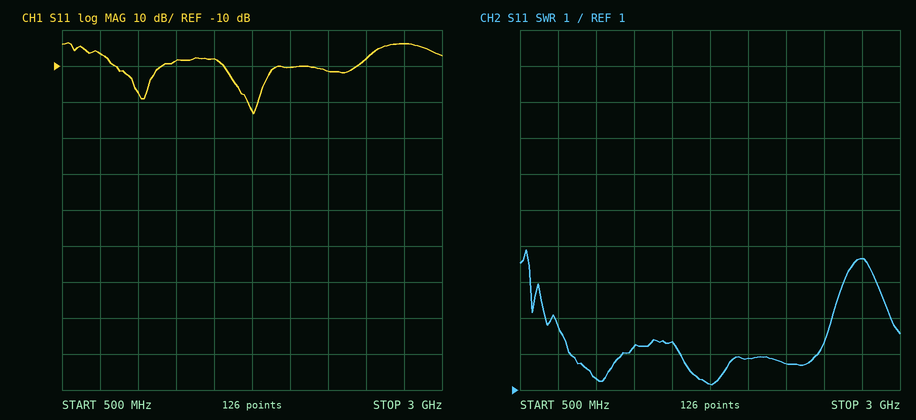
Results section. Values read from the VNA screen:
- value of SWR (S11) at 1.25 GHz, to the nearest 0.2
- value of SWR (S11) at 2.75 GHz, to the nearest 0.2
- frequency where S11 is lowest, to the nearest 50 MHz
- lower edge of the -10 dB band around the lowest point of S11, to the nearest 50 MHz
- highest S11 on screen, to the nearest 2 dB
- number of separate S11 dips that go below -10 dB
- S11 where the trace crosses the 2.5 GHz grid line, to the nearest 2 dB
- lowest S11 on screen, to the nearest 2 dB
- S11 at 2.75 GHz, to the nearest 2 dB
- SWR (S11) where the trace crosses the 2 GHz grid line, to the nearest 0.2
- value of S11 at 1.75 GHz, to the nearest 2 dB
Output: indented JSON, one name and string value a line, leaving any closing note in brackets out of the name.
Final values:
{
  "value of SWR (S11) at 1.25 GHz, to the nearest 0.2": "2.2",
  "value of SWR (S11) at 2.75 GHz, to the nearest 0.2": "4.6",
  "frequency where S11 is lowest, to the nearest 50 MHz": "1.75 GHz",
  "lower edge of the -10 dB band around the lowest point of S11, to the nearest 50 MHz": "1.55 GHz",
  "highest S11 on screen, to the nearest 2 dB": "-4 dB",
  "number of separate S11 dips that go below -10 dB": "2",
  "S11 where the trace crosses the 2.5 GHz grid line, to the nearest 2 dB": "-8 dB",
  "lowest S11 on screen, to the nearest 2 dB": "-24 dB",
  "S11 at 2.75 GHz, to the nearest 2 dB": "-4 dB",
  "SWR (S11) where the trace crosses the 2 GHz grid line, to the nearest 0.2": "1.8",
  "value of S11 at 1.75 GHz, to the nearest 2 dB": "-22 dB"
}
